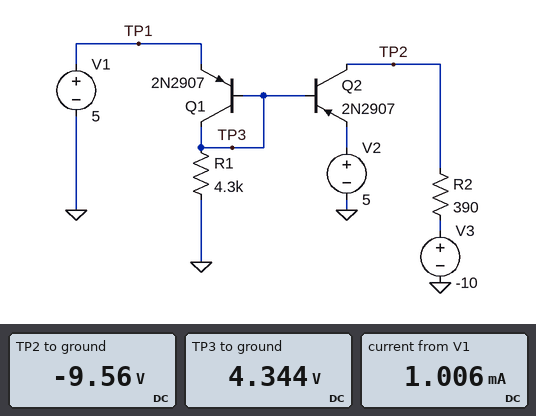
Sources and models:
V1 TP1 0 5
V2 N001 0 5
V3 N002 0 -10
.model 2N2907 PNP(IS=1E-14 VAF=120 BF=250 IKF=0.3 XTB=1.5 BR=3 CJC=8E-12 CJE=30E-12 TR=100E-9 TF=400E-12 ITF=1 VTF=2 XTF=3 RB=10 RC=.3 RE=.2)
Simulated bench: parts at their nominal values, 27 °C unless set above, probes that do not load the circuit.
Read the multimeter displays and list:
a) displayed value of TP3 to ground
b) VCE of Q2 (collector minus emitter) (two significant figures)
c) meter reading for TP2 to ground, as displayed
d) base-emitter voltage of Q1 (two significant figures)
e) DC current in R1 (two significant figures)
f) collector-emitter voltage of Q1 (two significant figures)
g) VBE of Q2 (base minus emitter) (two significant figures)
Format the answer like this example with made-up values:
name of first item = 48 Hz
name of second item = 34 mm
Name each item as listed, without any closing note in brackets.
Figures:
displayed value of TP3 to ground = 4.344 V
VCE of Q2 (collector minus emitter) = -15 V
meter reading for TP2 to ground, as displayed = -9.56 V
base-emitter voltage of Q1 = -660 mV
DC current in R1 = 1.0 mA
collector-emitter voltage of Q1 = -660 mV
VBE of Q2 (base minus emitter) = -660 mV
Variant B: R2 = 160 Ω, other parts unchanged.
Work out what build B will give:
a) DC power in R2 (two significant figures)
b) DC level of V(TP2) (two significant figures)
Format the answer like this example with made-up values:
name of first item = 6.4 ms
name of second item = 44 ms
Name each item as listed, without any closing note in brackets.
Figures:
DC power in R2 = 200 µW
DC level of V(TP2) = -9.8 V
